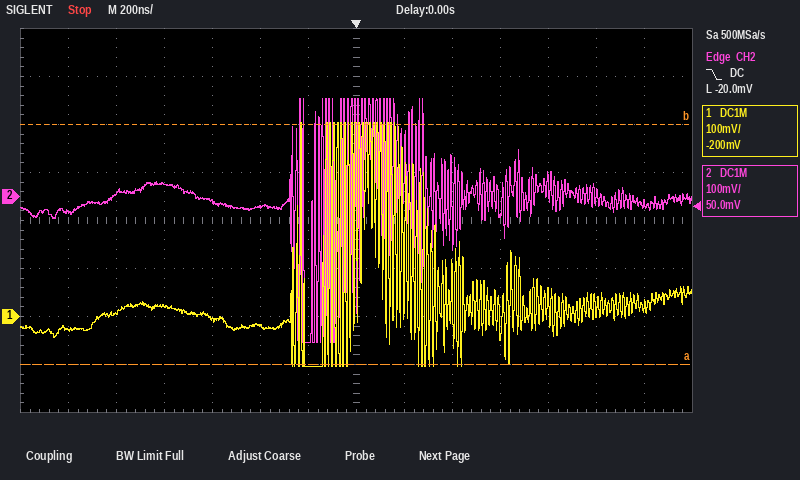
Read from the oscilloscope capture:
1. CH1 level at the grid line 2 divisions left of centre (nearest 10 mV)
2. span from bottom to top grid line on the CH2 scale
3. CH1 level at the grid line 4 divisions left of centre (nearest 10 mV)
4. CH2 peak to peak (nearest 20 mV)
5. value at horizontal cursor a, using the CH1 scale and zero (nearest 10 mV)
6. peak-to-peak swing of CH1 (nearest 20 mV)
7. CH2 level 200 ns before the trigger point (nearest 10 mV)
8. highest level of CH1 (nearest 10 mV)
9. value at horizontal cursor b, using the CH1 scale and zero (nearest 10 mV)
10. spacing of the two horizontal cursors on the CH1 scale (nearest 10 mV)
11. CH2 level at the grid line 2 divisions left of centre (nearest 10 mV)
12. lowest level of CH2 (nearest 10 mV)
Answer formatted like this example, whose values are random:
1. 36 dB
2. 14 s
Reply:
1. -20 mV
2. 800 mV
3. 20 mV
4. 500 mV
5. -100 mV
6. 500 mV
7. -300 mV
8. 400 mV
9. 400 mV
10. 500 mV
11. -20 mV
12. -300 mV
